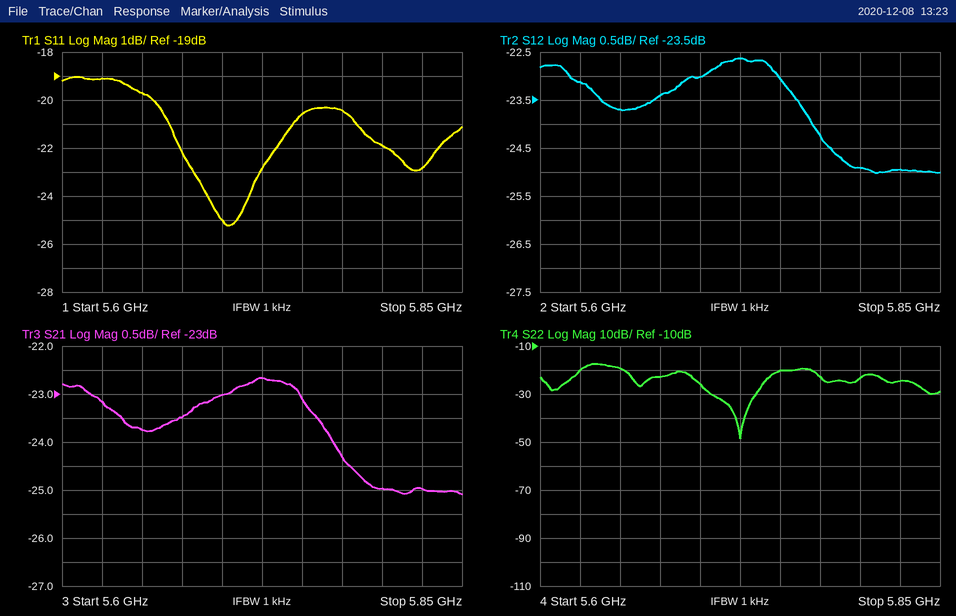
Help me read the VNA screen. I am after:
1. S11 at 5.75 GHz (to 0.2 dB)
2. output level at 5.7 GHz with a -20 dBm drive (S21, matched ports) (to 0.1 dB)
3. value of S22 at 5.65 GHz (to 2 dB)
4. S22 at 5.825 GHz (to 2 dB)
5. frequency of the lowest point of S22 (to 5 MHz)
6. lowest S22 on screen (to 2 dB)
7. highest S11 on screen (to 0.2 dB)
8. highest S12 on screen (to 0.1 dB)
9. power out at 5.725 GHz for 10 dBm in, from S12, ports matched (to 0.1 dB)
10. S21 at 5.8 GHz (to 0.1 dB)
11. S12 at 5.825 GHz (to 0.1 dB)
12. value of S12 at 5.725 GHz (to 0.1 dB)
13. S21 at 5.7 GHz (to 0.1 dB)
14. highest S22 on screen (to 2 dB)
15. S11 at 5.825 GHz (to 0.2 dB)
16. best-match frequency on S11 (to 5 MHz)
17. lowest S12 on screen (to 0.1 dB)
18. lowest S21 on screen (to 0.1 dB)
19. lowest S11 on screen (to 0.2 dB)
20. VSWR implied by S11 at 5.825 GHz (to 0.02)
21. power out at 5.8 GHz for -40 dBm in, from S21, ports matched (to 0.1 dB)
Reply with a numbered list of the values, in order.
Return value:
1. -20.6 dB
2. -43.0 dBm
3. -20 dB
4. -24 dB
5. 5.725 GHz
6. -48 dB
7. -19.0 dB
8. -22.6 dB
9. -12.6 dBm
10. -25.0 dB
11. -24.9 dB
12. -22.6 dB
13. -23.0 dB
14. -18 dB
15. -22.8 dB
16. 5.705 GHz
17. -25.0 dB
18. -25.1 dB
19. -25.2 dB
20. 1.16
21. -65.0 dBm
